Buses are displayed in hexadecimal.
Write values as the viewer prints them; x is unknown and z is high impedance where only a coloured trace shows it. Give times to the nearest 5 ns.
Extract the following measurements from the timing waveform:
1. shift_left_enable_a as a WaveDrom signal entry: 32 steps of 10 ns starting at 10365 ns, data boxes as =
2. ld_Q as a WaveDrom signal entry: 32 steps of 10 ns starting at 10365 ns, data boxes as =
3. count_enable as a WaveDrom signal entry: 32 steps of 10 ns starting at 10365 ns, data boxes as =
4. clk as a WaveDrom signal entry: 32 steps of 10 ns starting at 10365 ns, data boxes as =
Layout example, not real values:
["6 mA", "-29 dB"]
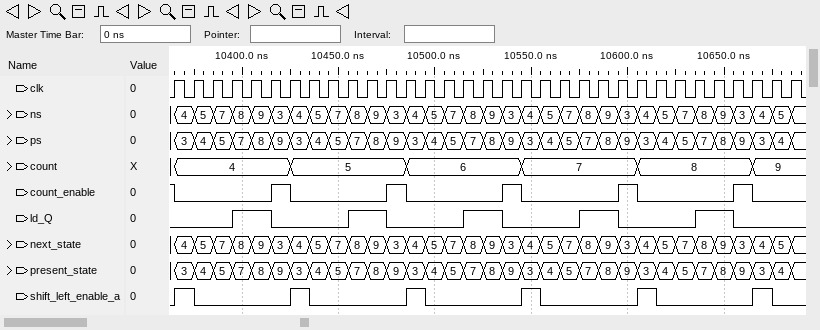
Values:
["{name: 'shift_left_enable_a', wave: '10....10....10....10....10....10'}", "{name: 'ld_Q', wave: '0..1.0...1.0...1.0...1.0...1.0..'}", "{name: 'count_enable', wave: '0....10....10....10....10....10.'}", "{name: 'clk', wave: 'p...............................'}"]
